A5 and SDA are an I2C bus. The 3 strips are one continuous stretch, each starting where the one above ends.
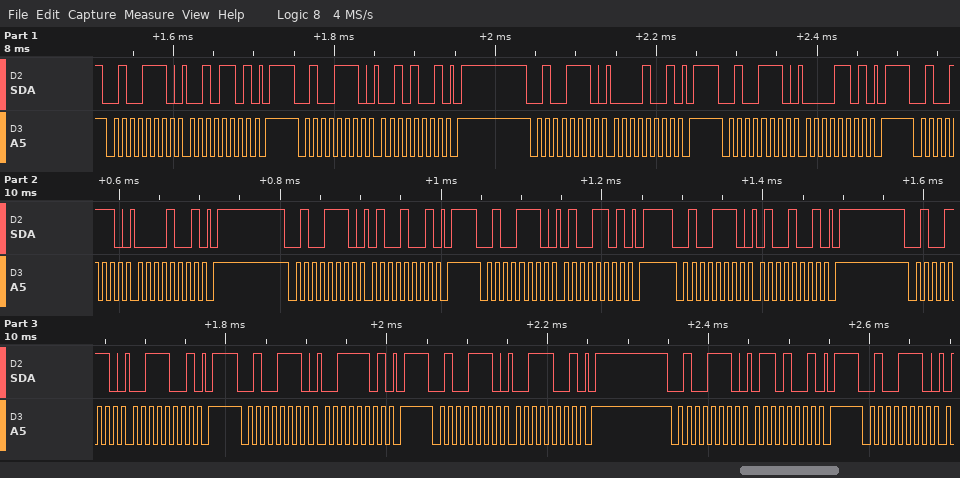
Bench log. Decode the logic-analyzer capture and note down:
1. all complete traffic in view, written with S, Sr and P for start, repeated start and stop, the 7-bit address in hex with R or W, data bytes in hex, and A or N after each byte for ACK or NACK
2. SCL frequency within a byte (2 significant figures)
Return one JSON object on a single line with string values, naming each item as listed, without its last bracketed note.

{"all complete traffic in view, written with S, Sr and P for start, repeated start and stop, the 7-bit address in hex with R or W, data bytes in hex, and A or N after each byte for ACK or NACK": "S 27W A 2D A P S 27W A 29 A P S 27W A 09 A P S 27W A 0D A P S 27W A 09 A P S 27W A 49 A P S 27W A 4D A P S 27W A 49 A P S 27W A 39 A P S 27W A 3D A P S 27W A 39 A P S 27W A 69 A P S 27W A", "SCL frequency within a byte": "100 kHz"}
